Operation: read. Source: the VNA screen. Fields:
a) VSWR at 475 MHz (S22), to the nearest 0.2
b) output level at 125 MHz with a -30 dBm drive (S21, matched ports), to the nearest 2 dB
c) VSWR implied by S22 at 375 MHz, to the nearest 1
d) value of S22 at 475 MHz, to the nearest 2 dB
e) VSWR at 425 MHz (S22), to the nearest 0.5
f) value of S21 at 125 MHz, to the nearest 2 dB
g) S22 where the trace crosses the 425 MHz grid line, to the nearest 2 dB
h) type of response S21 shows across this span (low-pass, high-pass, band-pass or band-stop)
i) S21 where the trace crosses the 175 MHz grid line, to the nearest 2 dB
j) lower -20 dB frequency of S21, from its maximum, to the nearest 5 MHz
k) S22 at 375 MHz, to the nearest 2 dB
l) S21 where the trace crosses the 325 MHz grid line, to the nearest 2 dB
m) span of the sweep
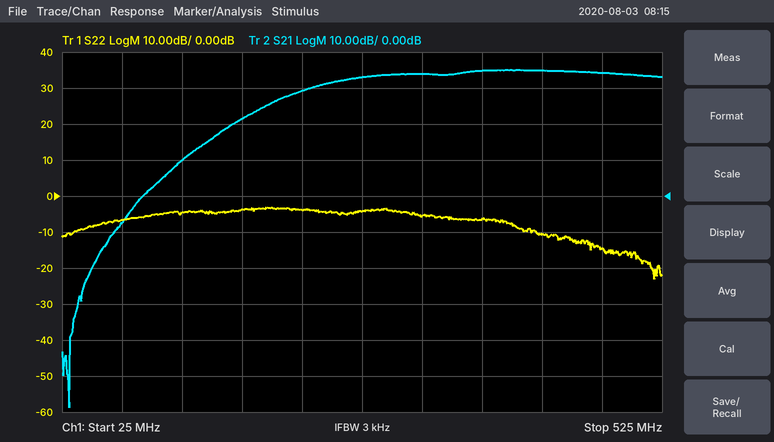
1.4
-20 dBm
3
-14 dB
2.0
10 dB
-10 dB
high-pass
22 dB
145 MHz
-6 dB
34 dB
500 MHz
